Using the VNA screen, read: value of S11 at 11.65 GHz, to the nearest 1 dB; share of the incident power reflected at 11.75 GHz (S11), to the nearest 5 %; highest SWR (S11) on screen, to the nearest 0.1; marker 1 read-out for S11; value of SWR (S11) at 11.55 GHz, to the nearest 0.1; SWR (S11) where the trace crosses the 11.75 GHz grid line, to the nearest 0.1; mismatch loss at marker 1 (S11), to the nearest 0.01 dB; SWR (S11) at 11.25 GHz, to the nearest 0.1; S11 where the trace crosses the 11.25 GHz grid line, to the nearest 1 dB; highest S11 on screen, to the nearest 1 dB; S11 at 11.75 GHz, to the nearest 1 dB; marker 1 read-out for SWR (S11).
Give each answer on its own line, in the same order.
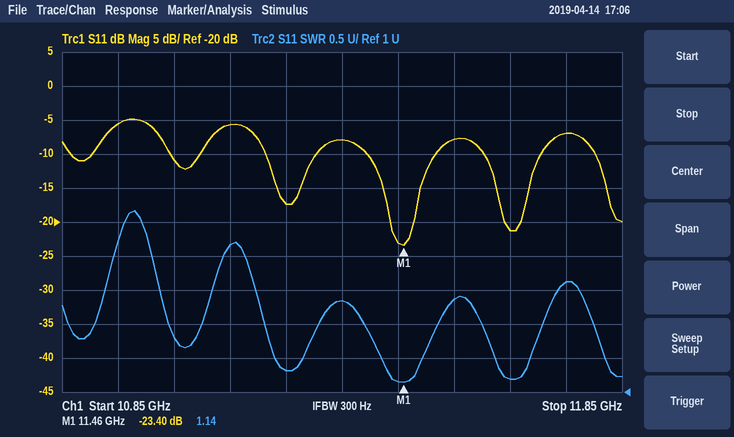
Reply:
-21 dB
20 %
3.7
-23.40 dB
2.4
2.6
0.02 dB
1.3
-17 dB
-5 dB
-7 dB
1.14
